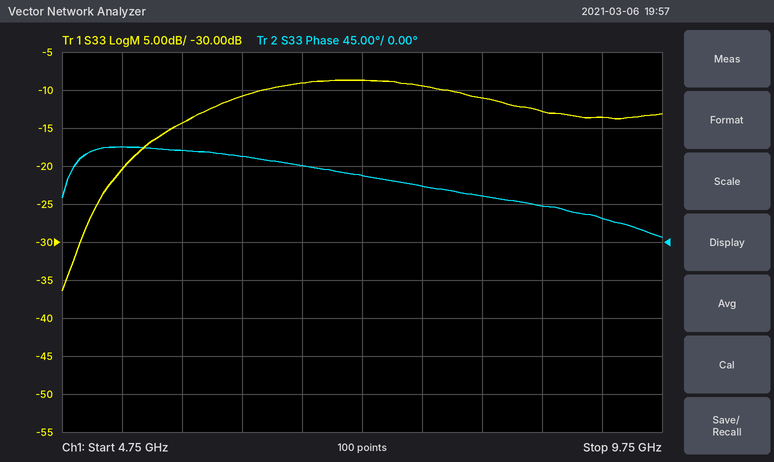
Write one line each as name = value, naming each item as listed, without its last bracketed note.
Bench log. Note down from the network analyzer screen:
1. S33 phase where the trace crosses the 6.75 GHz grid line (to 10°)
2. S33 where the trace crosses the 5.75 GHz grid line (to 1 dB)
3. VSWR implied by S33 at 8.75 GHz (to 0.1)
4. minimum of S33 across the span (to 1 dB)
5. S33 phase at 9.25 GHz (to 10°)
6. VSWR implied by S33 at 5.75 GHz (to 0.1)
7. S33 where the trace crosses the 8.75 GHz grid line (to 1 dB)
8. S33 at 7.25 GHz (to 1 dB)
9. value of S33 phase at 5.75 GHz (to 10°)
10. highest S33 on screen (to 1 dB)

S33 phase where the trace crosses the 6.75 GHz grid line = 90°
S33 where the trace crosses the 5.75 GHz grid line = -14 dB
VSWR implied by S33 at 8.75 GHz = 1.6
minimum of S33 across the span = -36 dB
S33 phase at 9.25 GHz = 30°
VSWR implied by S33 at 5.75 GHz = 1.5
S33 where the trace crosses the 8.75 GHz grid line = -13 dB
S33 at 7.25 GHz = -9 dB
value of S33 phase at 5.75 GHz = 110°
highest S33 on screen = -9 dB
